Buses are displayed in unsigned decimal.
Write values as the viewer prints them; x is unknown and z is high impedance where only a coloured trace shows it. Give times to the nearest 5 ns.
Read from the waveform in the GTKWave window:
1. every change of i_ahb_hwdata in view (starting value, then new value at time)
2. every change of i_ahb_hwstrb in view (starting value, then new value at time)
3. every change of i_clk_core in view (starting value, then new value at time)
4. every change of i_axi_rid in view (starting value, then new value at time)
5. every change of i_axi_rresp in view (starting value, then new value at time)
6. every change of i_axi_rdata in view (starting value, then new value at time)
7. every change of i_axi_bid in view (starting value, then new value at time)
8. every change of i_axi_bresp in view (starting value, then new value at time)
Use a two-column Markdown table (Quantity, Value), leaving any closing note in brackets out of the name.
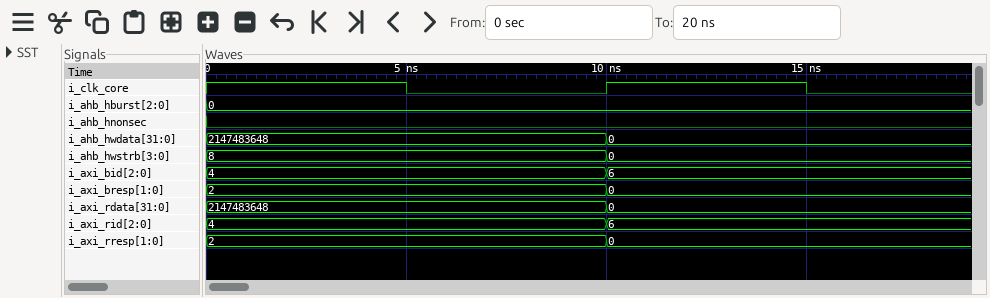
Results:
| Quantity | Value |
|---|---|
| every change of i_ahb_hwdata in view | 2147483648, 0 at 10 ns |
| every change of i_ahb_hwstrb in view | 8, 0 at 10 ns |
| every change of i_clk_core in view | 1, 0 at 5 ns, 1 at 10 ns, 0 at 15 ns |
| every change of i_axi_rid in view | 4, 6 at 10 ns |
| every change of i_axi_rresp in view | 2, 0 at 10 ns |
| every change of i_axi_rdata in view | 2147483648, 0 at 10 ns |
| every change of i_axi_bid in view | 4, 6 at 10 ns |
| every change of i_axi_bresp in view | 2, 0 at 10 ns |
